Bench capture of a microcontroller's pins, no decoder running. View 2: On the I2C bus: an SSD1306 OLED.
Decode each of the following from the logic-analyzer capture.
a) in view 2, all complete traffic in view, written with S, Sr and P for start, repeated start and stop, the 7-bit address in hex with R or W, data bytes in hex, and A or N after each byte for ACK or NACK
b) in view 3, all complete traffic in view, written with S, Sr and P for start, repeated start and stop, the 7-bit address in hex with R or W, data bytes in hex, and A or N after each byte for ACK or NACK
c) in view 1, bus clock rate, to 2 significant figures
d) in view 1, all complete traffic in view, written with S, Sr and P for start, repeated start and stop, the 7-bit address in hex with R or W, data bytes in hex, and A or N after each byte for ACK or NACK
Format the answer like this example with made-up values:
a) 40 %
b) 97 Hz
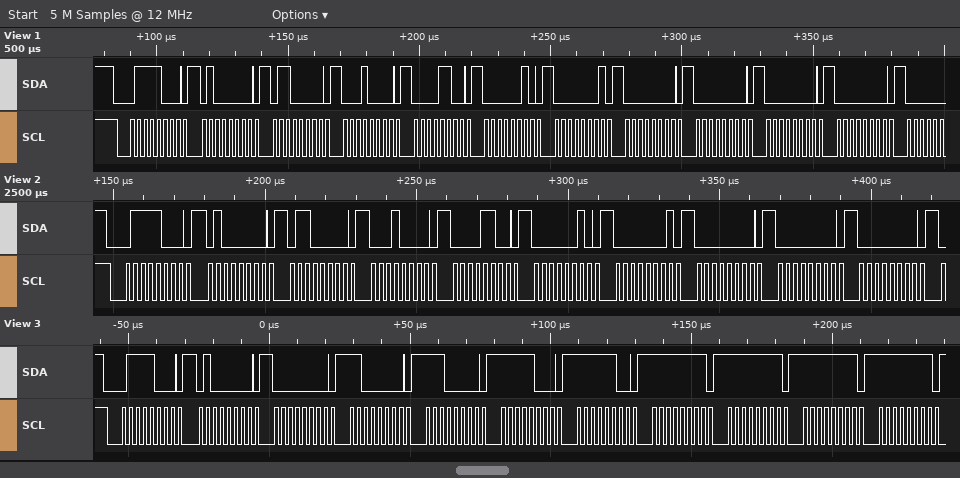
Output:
a) S 3CW A 40 A 60 A 10 A 0C A 02 A 01 A 00 A 00 A 00 A
b) S 3CW A 40 A 00 A C0 A E0 A F8 A FC A FF A FF A FF A FF A
c) 400 kHz
d) S 3CW A 40 A 60 A 10 A 0C A 02 A 01 A 00 A 00 A 00 A 00 A
